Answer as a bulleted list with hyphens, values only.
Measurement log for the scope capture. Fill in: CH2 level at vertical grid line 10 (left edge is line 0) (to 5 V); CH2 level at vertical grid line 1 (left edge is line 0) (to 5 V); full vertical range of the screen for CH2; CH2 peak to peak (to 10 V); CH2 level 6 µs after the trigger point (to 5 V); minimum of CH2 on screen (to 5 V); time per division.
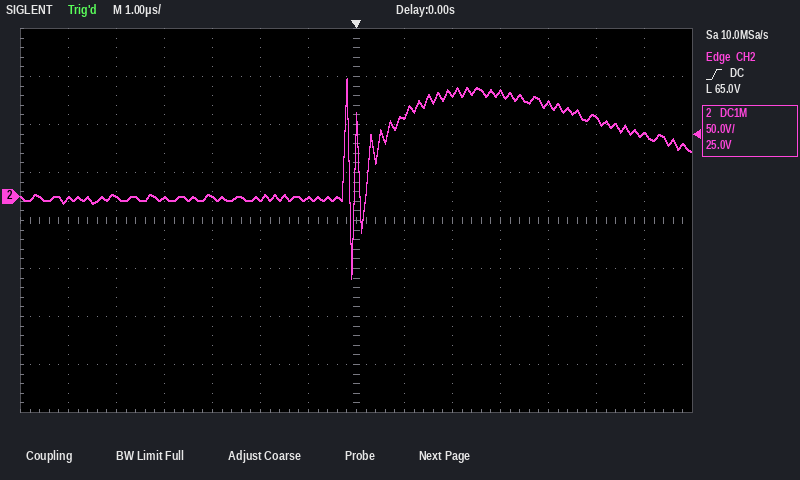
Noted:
- 110 V
- 0 V
- 400 V
- 210 V
- 65 V
- -85 V
- 1 µs
